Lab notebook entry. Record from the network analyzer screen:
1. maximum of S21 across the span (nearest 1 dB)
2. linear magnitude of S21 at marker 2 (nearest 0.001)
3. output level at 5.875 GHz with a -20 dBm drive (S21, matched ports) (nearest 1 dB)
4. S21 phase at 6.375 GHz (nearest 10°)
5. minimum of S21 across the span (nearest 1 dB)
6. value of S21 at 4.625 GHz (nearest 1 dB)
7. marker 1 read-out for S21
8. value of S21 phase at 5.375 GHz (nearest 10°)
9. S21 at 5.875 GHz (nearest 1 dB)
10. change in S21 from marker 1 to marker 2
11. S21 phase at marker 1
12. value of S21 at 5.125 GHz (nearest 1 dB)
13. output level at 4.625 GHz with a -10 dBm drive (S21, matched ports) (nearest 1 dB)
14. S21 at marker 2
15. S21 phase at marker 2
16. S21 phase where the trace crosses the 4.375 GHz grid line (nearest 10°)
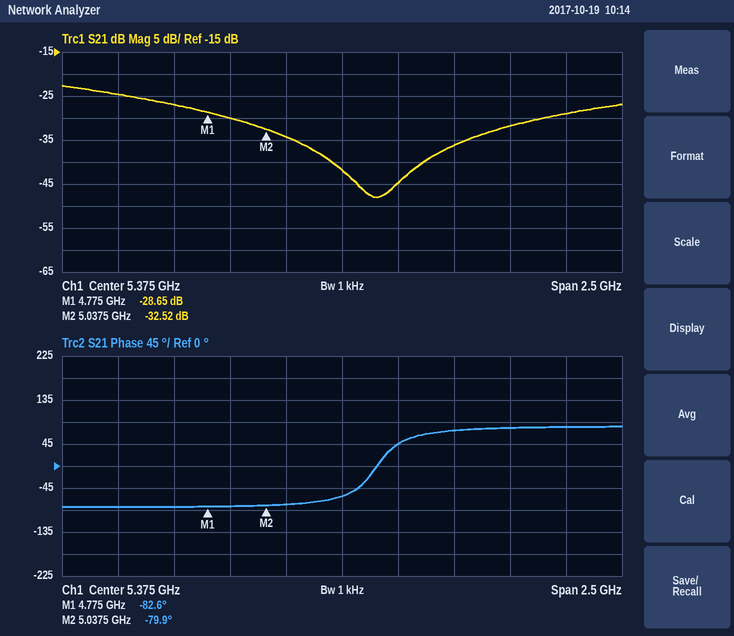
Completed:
-23 dB
0.024
-56 dBm
80°
-48 dB
-27 dB
-28.65 dB
-60°
-36 dB
-3.87 dB
-82.6°
-34 dB
-37 dBm
-32.52 dB
-79.9°
-80°
